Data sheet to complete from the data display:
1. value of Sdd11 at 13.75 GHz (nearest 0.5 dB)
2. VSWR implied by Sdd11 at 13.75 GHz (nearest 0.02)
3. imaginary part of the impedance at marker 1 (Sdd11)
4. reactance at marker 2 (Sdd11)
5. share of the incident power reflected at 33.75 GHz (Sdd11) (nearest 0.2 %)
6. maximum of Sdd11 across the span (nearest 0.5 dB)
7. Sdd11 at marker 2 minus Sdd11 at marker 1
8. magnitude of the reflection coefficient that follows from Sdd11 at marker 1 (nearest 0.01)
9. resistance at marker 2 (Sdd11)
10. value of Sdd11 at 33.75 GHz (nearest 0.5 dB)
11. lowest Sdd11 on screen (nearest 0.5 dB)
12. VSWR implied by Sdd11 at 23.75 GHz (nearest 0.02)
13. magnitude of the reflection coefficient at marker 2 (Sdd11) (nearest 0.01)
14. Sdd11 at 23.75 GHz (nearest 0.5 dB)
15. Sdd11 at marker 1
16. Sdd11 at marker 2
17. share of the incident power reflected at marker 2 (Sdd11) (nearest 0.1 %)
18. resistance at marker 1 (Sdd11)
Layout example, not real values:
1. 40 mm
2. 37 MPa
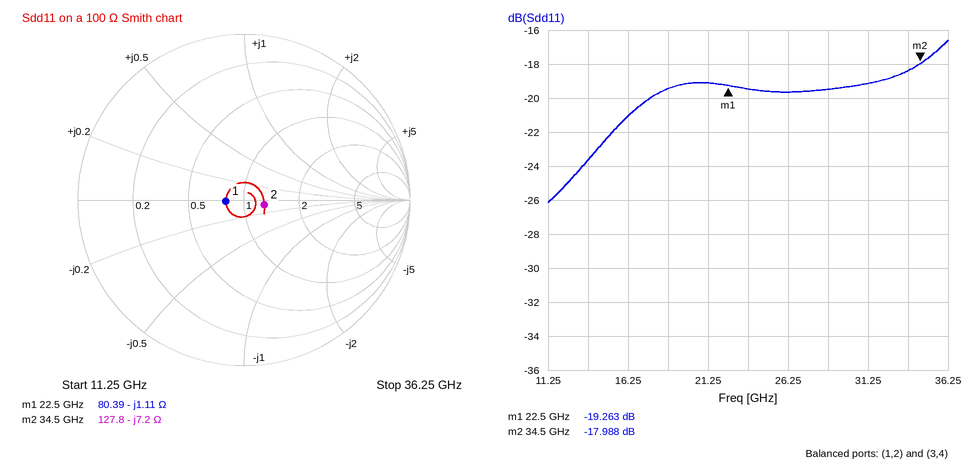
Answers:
1. -23.5 dB
2. 1.14
3. -1.11 Ω
4. -7.2 Ω
5. 1.4 %
6. -16.5 dB
7. 1.275 dB
8. 0.11
9. 127.8 Ω
10. -18.5 dB
11. -26.0 dB
12. 1.24
13. 0.13
14. -19.5 dB
15. -19.263 dB
16. -17.988 dB
17. 1.6 %
18. 80.39 Ω
